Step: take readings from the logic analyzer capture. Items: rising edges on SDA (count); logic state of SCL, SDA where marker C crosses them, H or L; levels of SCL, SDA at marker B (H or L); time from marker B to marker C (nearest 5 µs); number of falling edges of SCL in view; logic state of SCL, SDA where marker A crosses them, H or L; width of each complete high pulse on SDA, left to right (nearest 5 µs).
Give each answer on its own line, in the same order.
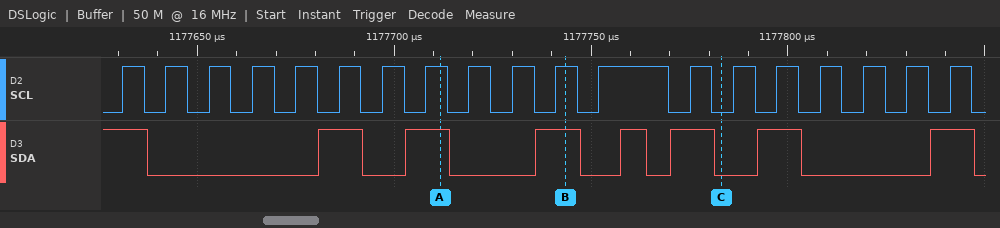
7
SCL=L, SDA=L
SCL=H, SDA=H
40 µs
19
SCL=H, SDA=H
10 µs, 10 µs, 10 µs, 5 µs, 10 µs, 10 µs, 10 µs
